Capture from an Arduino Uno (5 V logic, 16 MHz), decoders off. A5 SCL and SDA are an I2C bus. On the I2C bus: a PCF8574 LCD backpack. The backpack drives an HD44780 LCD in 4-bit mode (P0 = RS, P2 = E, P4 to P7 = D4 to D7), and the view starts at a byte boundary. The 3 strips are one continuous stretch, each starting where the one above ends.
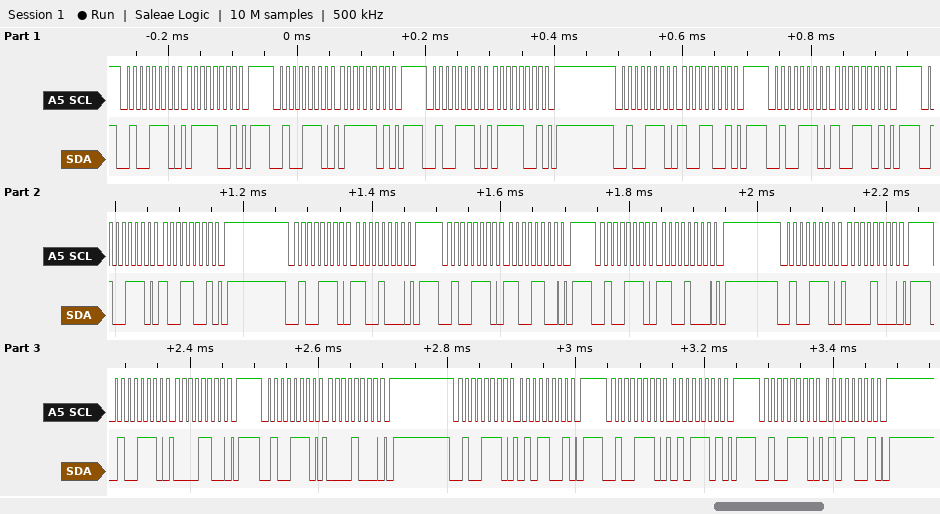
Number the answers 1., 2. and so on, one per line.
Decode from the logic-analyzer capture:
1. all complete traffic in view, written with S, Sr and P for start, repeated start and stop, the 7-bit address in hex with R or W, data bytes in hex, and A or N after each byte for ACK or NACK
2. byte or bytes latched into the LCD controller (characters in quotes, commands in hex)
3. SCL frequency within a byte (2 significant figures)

1. S 27W A 79 A P S 27W A 7D A P S 27W A 79 A P S 27W A 99 A P S 27W A 9D A P S 27W A 99 A P S 27W A C8 A P S 27W A CC A P S 27W A C8 A P S 27W A 08 A P S 27W A 0C A P S 27W A 08 A P S 27W A 59 A P S 27W A 5D A P S 27W A 59 A P
2. 'y' 0xC0
3. 100 kHz
